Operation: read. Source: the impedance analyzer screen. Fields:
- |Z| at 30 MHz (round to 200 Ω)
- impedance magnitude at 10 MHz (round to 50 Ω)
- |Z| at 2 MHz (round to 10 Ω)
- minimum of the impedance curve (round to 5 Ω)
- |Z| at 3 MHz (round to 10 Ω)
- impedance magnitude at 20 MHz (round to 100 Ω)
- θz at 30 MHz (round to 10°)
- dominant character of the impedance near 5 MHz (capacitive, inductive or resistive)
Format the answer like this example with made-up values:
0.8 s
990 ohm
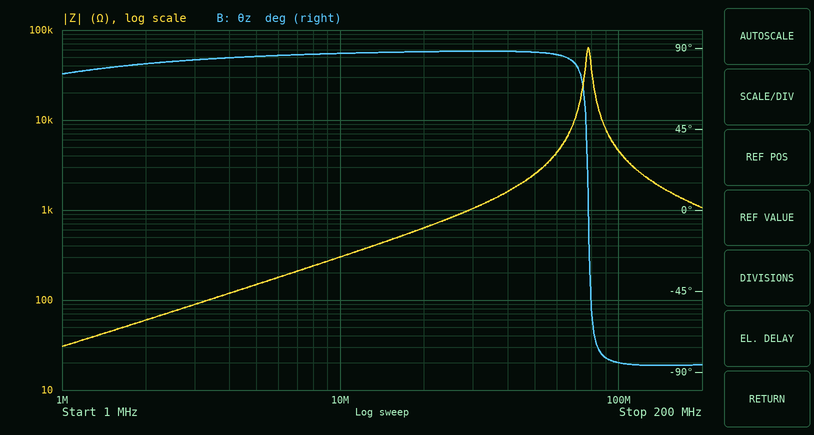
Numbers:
1.0 kΩ
300 Ω
60 Ω
30 Ω
90 Ω
600 Ω
90°
inductive
